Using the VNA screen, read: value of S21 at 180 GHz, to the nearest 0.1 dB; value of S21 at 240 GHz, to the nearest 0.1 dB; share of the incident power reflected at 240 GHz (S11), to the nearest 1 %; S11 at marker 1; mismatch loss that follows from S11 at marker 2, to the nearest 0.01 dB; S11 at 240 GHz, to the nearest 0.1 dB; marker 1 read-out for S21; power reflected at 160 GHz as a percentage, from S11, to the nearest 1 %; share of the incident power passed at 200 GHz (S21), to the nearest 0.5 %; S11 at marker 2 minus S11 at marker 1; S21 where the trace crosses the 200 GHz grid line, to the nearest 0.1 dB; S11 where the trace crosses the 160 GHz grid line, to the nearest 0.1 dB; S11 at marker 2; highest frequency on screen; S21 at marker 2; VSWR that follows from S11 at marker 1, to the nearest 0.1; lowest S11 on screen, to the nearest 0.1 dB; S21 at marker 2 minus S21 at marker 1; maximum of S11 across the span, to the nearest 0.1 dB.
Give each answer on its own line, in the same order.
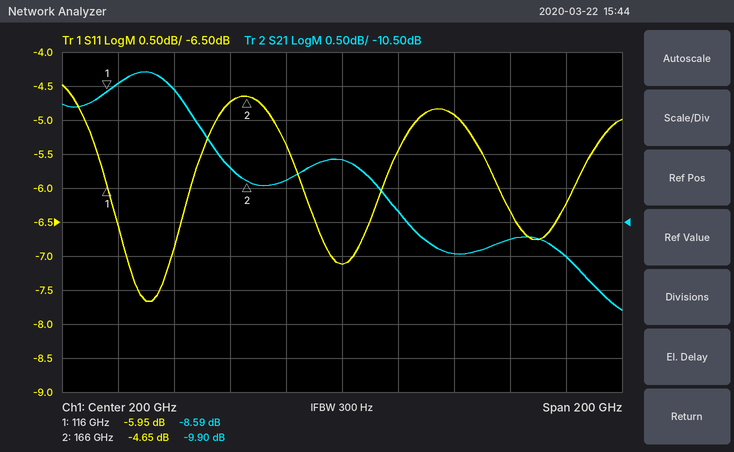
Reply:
-9.9 dB
-11.0 dB
32 %
-5.95 dB
1.82 dB
-4.9 dB
-8.59 dB
34 %
11.0 %
1.30 dB
-9.6 dB
-4.7 dB
-4.65 dB
300 GHz
-9.90 dB
3.0
-7.7 dB
-1.31 dB
-4.5 dB
